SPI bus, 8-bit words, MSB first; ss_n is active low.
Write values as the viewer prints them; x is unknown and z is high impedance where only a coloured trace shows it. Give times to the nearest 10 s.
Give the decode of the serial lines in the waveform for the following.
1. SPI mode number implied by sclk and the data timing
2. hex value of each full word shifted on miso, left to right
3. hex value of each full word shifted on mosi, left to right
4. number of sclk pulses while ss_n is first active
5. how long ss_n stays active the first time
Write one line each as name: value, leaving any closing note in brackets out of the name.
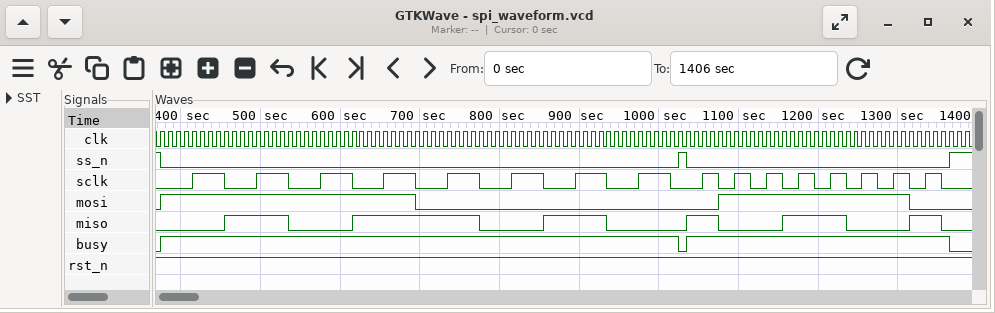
SPI mode number implied by sclk and the data timing: 0
hex value of each full word shifted on miso, left to right: 5A, 99
hex value of each full word shifted on mosi, left to right: F0, 7E
number of sclk pulses while ss_n is first active: 8
how long ss_n stays active the first time: 650 s
